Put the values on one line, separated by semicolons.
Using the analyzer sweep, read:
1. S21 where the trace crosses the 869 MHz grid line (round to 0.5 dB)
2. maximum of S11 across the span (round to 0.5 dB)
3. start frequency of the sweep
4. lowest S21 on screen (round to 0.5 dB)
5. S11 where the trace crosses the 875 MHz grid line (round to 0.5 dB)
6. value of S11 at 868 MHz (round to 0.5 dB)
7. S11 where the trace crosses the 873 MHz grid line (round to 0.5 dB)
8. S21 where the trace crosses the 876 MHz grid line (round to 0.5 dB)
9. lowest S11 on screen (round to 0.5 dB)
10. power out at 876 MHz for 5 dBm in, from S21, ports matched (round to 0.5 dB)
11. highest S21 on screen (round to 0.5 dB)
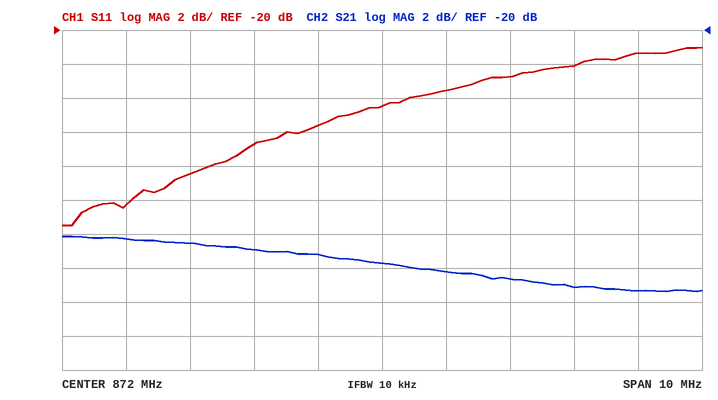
-32.5 dB; -21.0 dB; 867 MHz; -35.5 dB; -22.0 dB; -30.5 dB; -23.5 dB; -35.5 dB; -31.5 dB; -30.5 dBm; -32.0 dB
